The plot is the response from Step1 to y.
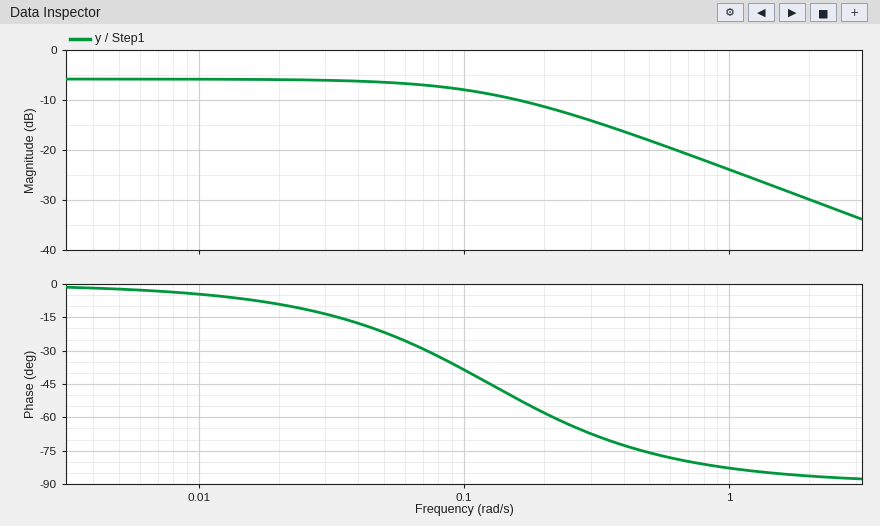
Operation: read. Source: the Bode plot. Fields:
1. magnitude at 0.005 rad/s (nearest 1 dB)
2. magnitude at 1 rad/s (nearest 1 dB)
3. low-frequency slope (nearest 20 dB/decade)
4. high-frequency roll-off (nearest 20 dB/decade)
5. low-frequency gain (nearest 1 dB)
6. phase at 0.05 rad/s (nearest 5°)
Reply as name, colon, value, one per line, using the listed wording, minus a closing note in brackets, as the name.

magnitude at 0.005 rad/s: -6 dB
magnitude at 1 rad/s: -24 dB
low-frequency slope: 0 dB/decade
high-frequency roll-off: -20 dB/decade
low-frequency gain: -6 dB
phase at 0.05 rad/s: -20°
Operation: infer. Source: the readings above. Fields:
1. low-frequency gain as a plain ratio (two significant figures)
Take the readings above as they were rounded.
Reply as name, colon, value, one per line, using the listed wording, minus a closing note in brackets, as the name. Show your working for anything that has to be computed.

low-frequency gain as a plain ratio: 10^(-6 / 20) = 0.50
